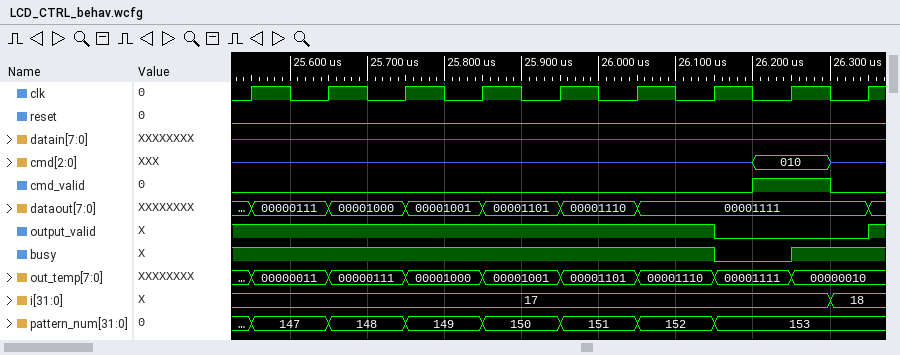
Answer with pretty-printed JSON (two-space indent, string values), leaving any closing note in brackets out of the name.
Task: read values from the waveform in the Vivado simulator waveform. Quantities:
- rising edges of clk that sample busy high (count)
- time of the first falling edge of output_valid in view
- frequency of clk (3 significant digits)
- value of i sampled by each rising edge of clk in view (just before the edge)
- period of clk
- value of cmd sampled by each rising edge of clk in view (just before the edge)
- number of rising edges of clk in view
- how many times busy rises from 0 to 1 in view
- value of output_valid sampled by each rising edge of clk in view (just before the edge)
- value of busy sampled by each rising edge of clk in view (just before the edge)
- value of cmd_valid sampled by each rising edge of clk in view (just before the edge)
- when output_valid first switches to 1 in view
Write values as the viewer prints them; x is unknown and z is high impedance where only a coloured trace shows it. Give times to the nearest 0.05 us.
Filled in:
{
  "rising edges of clk that sample busy high": "8",
  "time of the first falling edge of output_valid in view": "26.15 us",
  "frequency of clk": "10.0 MHz",
  "value of i sampled by each rising edge of clk in view": "17, 17, 17, 17, 17, 17, 17, 17, 18",
  "period of clk": "0.1 us",
  "value of cmd sampled by each rising edge of clk in view": "z, z, z, z, z, z, z, 010, z",
  "number of rising edges of clk in view": "9",
  "how many times busy rises from 0 to 1 in view": "1",
  "value of output_valid sampled by each rising edge of clk in view": "1 1 1 1 1 1 1 0 0",
  "value of busy sampled by each rising edge of clk in view": "1 1 1 1 1 1 1 0 1",
  "value of cmd_valid sampled by each rising edge of clk in view": "0 0 0 0 0 0 0 1 0",
  "when output_valid first switches to 1 in view": "26.35 us"
}
